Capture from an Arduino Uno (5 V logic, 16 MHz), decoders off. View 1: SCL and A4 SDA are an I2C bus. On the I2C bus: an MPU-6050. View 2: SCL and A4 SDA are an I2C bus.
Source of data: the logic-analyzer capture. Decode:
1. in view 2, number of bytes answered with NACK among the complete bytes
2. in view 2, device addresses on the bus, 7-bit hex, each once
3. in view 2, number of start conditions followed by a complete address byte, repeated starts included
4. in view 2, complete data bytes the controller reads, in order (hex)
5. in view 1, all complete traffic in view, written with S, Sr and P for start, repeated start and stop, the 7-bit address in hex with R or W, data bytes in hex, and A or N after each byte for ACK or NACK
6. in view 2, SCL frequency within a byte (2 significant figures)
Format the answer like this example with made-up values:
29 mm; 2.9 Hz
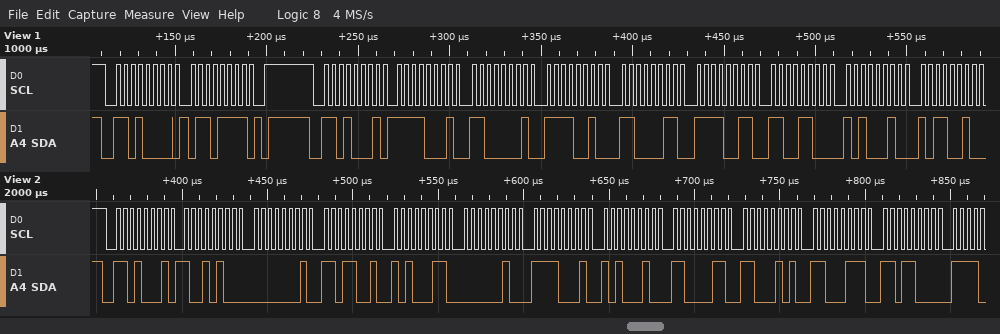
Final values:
0; 0x68; 1; 94 01 D9 A3 02 F1 A2 C3 C5 C7 D8; S 68W A 6F A P S 68R A F1 A C1 A F2 A C3 A F3 A CC A A2 A B2 A; 250 kHz
